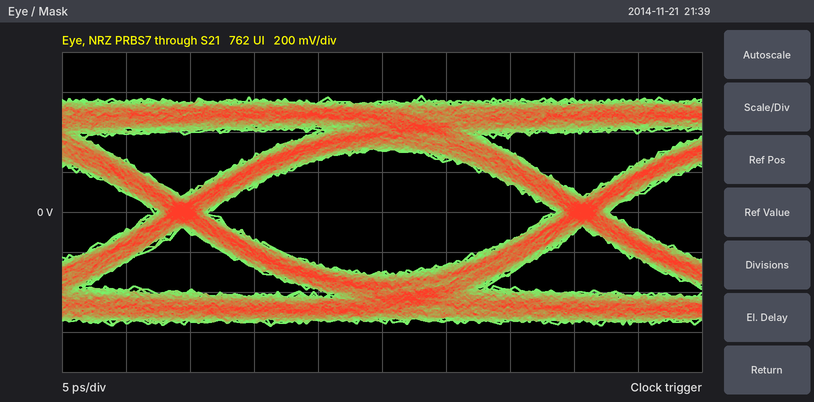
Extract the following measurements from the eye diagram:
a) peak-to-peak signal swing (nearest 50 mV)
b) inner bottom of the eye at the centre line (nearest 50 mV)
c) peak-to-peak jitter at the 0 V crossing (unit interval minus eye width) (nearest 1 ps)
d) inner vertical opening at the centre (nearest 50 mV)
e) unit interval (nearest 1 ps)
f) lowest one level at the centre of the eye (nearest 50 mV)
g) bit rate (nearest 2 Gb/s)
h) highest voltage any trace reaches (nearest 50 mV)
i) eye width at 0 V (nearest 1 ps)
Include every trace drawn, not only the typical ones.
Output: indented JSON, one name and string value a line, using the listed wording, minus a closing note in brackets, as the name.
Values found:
{
  "peak-to-peak signal swing": "1.15 V",
  "inner bottom of the eye at the centre line": "-300 mV",
  "peak-to-peak jitter at the 0 V crossing (unit interval minus eye width)": "4 ps",
  "inner vertical opening at the centre": "600 mV",
  "unit interval": "31 ps",
  "lowest one level at the centre of the eye": "300 mV",
  "bit rate": "32 Gb/s",
  "highest voltage any trace reaches": "600 mV",
  "eye width at 0 V": "27 ps"
}
